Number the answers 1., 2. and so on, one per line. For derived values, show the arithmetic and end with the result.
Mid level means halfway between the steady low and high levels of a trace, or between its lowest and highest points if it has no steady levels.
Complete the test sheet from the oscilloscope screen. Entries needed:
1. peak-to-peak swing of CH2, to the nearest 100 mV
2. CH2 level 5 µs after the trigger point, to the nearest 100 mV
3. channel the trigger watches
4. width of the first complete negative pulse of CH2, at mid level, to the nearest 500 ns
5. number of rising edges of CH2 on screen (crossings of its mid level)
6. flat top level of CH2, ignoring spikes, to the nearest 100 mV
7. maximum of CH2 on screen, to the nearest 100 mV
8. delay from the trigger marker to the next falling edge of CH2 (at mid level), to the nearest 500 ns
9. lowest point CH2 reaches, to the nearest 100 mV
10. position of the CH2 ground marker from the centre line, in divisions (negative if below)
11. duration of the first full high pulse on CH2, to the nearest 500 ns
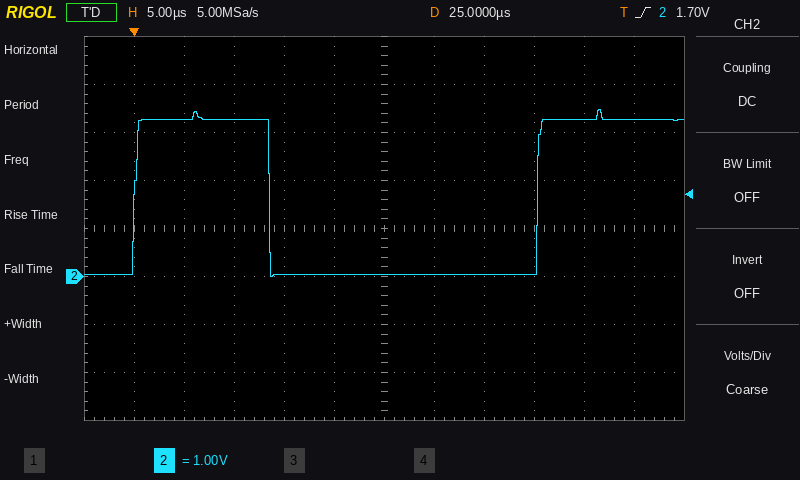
1. 3.5 V − (0.0 V) = 3.5 V
2. 3.3 V
3. CH2
4. 27.0 µs
5. 2
6. 3.3 V
7. 3.5 V
8. 13.5 µs
9. 0.0 V
10. -1.0 div
11. 13.5 µs
